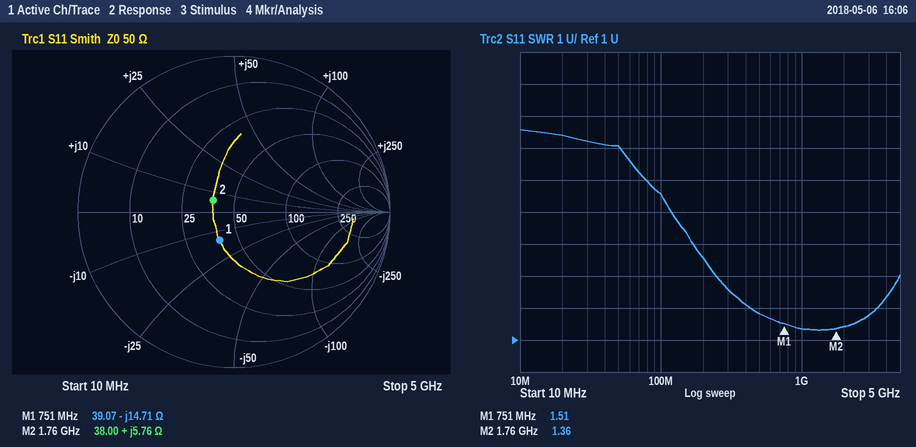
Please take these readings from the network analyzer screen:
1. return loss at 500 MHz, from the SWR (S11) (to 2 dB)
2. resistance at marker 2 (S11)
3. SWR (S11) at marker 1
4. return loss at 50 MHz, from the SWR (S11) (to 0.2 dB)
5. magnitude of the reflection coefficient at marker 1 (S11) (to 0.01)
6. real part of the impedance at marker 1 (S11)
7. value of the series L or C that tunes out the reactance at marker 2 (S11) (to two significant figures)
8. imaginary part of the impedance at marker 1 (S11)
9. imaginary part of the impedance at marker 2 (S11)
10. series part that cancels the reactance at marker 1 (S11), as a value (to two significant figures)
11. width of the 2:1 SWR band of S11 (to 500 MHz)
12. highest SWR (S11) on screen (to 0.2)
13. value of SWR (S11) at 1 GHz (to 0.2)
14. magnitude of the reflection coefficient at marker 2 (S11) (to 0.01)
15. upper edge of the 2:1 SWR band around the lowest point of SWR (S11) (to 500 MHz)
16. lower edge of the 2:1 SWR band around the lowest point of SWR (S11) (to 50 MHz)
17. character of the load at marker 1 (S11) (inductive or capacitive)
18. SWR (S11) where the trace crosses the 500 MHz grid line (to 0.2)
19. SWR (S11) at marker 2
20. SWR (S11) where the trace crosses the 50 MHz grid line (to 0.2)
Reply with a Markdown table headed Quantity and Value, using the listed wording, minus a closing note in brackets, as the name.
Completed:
| Quantity | Value |
|---|---|
| return loss at 500 MHz, from the SWR (S11) | 10 dB |
| resistance at marker 2 | 38.00 Ω |
| SWR (S11) at marker 1 | 1.51 |
| return loss at 50 MHz, from the SWR (S11) | 2.4 dB |
| magnitude of the reflection coefficient at marker 1 (S11) | 0.20 |
| real part of the impedance at marker 1 | 39.07 Ω |
| value of the series L or C that tunes out the reactance at marker 2 (S11) | 16 pF |
| imaginary part of the impedance at marker 1 | -14.71 Ω |
| imaginary part of the impedance at marker 2 | +5.76 Ω |
| series part that cancels the reactance at marker 1 (S11), as a value | 3.1 nH |
| width of the 2:1 SWR band of S11 | 3.0 GHz |
| highest SWR (S11) on screen | 7.6 |
| value of SWR (S11) at 1 GHz | 1.4 |
| magnitude of the reflection coefficient at marker 2 (S11) | 0.15 |
| upper edge of the 2:1 SWR band around the lowest point of SWR (S11) | 3.5 GHz |
| lower edge of the 2:1 SWR band around the lowest point of SWR (S11) | 450 MHz |
| character of the load at marker 1 (S11) | capacitive |
| SWR (S11) where the trace crosses the 500 MHz grid line | 1.8 |
| SWR (S11) at marker 2 | 1.36 |
| SWR (S11) where the trace crosses the 50 MHz grid line | 7.0 |
